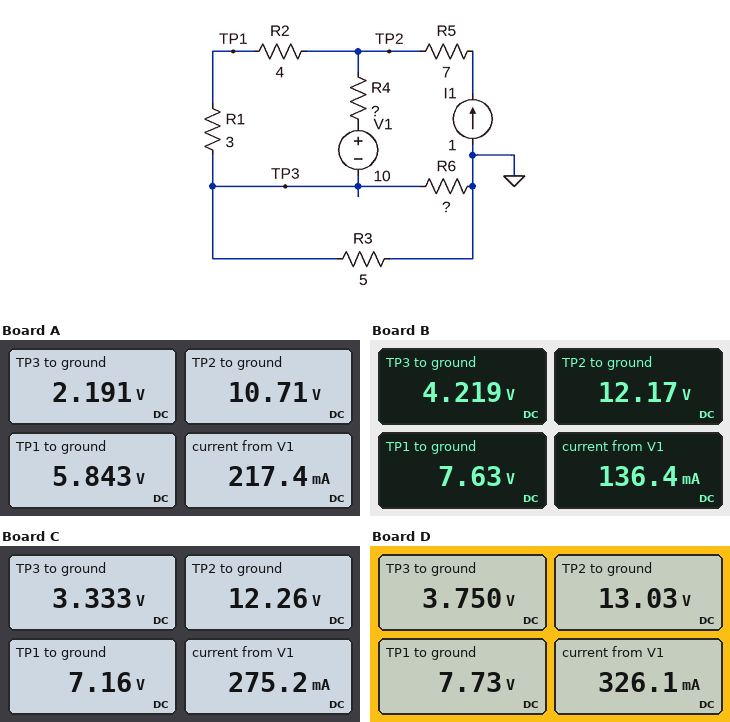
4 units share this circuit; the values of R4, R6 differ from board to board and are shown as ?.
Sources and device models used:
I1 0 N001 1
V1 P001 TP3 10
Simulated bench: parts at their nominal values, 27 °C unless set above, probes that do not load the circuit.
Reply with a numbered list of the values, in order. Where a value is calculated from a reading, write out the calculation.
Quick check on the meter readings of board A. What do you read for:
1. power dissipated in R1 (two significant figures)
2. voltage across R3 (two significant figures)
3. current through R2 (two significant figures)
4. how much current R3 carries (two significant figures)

1. (5.843 V - 2.191 V)^2 / 3 Ω = 4.4 W
2. 2.191 V = 2.2 V
3. (10.71 V - 5.843 V) / 4 Ω = 1.2 A
4. (2.191 V) / 5 Ω = 440 mA
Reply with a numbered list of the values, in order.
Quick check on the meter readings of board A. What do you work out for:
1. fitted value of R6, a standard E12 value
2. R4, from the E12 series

1. 3.9 Ω
2. 6.8 Ω
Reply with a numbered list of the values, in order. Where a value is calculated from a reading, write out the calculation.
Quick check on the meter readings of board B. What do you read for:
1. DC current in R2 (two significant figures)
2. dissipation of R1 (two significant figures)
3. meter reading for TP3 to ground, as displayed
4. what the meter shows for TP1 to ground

1. (12.17 V - 7.63 V) / 4 Ω = 1.1 A
2. (7.63 V - 4.219 V)^2 / 3 Ω = 3.9 W
3. 4.219 V
4. 7.63 V
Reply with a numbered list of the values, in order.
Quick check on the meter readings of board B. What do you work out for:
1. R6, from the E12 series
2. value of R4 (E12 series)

1. 27 Ω
2. 15 Ω
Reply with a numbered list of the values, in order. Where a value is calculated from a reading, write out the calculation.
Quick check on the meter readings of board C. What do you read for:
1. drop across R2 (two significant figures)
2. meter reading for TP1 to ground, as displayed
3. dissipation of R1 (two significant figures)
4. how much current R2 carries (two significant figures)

1. 12.26 V - 7.16 V = 5.1 V
2. 7.16 V
3. (7.16 V - 3.333 V)^2 / 3 Ω = 4.9 W
4. (12.26 V - 7.16 V) / 4 Ω = 1.3 A
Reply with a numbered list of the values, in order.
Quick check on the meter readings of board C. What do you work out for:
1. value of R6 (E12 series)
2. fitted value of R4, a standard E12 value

1. 10 Ω
2. 3.9 Ω
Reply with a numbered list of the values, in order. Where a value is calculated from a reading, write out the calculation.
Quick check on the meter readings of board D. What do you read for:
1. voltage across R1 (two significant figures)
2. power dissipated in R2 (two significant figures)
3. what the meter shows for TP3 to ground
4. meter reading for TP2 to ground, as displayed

1. 7.73 V - 3.75 V = 4.0 V
2. (13.03 V - 7.73 V)^2 / 4 Ω = 7.0 W
3. 3.750 V
4. 13.03 V
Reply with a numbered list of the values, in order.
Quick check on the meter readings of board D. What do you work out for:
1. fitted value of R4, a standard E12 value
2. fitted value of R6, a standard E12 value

1. 2.2 Ω
2. 15 Ω
